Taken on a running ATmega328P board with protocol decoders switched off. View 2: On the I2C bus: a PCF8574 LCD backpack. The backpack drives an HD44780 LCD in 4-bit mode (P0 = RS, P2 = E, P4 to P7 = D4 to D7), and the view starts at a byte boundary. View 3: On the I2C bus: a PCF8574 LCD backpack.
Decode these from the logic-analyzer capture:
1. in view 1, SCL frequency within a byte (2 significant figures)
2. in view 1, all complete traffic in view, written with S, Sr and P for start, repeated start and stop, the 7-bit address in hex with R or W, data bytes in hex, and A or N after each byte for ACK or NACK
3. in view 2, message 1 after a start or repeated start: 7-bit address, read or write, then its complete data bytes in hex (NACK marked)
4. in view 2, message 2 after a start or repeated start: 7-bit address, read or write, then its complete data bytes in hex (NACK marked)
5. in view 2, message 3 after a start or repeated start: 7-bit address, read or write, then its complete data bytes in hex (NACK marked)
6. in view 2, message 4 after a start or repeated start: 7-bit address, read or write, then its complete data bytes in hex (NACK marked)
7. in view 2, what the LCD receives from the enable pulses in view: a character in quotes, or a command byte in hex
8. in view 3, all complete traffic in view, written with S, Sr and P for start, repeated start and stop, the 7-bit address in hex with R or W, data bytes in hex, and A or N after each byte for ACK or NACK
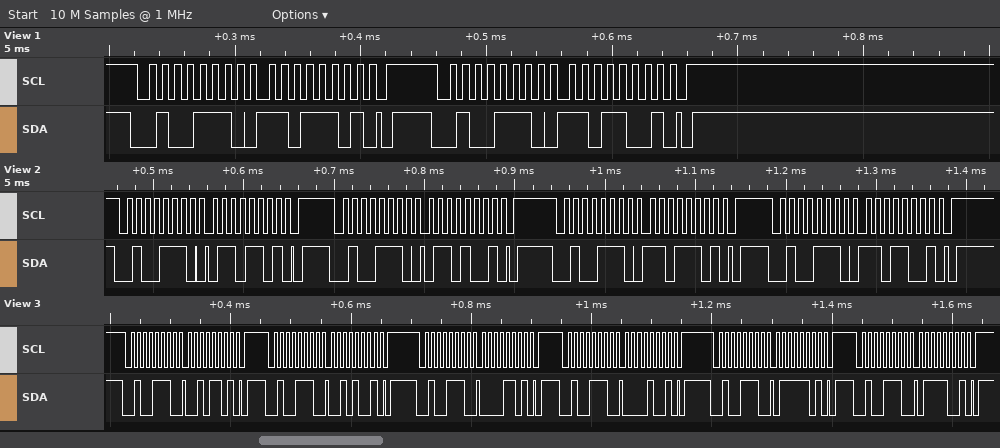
100 kHz
S 27W A DD A P S 27W A D9 A P
0x27 write: 6D
0x27 write: 69
0x27 write: DD
0x27 write: D9
'm'
S 27W A 2D A P S 27W A 29 A P S 27W A 0D A P S 27W A 09 A P S 27W A 7D A P S 27W A 79 A P
